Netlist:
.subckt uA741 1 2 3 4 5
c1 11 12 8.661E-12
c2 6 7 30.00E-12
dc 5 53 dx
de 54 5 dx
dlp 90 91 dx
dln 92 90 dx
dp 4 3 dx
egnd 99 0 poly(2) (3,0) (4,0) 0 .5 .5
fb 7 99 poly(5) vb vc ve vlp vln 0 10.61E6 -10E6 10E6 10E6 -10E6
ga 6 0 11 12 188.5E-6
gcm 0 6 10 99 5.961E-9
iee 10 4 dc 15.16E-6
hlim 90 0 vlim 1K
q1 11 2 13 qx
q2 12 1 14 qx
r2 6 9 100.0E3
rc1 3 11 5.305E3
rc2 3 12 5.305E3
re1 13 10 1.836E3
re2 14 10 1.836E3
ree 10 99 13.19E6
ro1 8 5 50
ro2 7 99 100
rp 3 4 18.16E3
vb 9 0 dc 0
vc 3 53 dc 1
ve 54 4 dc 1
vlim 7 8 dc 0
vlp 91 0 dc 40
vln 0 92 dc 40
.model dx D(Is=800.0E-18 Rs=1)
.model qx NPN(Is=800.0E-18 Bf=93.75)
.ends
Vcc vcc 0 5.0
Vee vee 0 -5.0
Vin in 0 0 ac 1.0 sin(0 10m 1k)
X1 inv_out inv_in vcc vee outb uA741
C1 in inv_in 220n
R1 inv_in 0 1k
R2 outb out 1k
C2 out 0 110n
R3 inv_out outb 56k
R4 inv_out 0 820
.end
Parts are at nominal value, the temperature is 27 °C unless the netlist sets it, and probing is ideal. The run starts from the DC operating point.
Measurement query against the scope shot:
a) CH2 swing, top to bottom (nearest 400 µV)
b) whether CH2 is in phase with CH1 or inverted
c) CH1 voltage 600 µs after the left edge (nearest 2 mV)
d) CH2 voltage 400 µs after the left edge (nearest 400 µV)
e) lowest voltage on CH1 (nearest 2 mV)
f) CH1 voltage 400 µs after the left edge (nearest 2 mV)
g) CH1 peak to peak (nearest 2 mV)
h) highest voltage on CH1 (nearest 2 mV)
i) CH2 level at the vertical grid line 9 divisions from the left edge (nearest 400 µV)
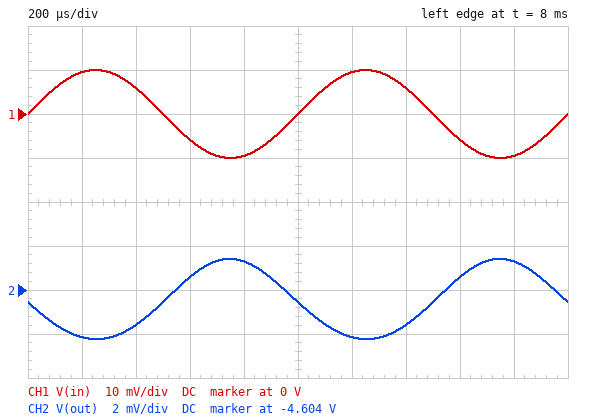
3.6 mV
inverted
-6 mV
-4.6056 V
-10 mV
6 mV
20 mV
10 mV
-4.6028 V
